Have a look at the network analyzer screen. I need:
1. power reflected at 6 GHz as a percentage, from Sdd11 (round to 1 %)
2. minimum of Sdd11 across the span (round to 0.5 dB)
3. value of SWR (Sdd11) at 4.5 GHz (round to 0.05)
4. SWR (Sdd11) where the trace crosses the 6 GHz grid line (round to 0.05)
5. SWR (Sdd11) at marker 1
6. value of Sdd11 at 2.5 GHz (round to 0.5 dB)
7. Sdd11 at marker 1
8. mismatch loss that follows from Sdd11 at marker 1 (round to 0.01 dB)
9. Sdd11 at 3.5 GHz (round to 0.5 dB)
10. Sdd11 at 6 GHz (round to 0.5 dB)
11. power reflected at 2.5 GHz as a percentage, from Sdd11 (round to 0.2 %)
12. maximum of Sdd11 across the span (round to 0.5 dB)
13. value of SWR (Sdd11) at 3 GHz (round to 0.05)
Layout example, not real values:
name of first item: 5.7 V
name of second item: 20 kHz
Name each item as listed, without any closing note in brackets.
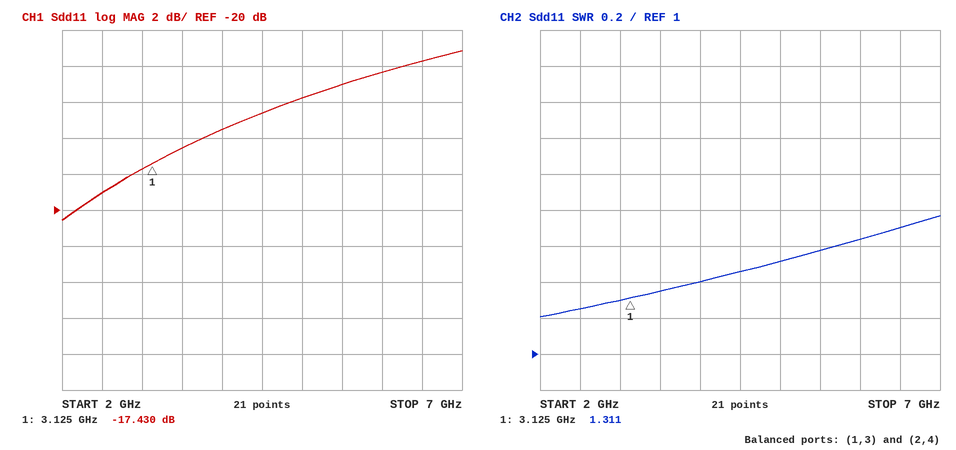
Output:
power reflected at 6 GHz as a percentage, from Sdd11: 6 %
minimum of Sdd11 across the span: -20.5 dB
value of SWR (Sdd11) at 4.5 GHz: 1.45
SWR (Sdd11) where the trace crosses the 6 GHz grid line: 1.65
SWR (Sdd11) at marker 1: 1.311
value of Sdd11 at 2.5 GHz: -19.0 dB
Sdd11 at marker 1: -17.430 dB
mismatch loss that follows from Sdd11 at marker 1: 0.08 dB
Sdd11 at 3.5 GHz: -16.5 dB
Sdd11 at 6 GHz: -12.5 dB
power reflected at 2.5 GHz as a percentage, from Sdd11: 1.2 %
maximum of Sdd11 across the span: -11.0 dB
value of SWR (Sdd11) at 3 GHz: 1.30
